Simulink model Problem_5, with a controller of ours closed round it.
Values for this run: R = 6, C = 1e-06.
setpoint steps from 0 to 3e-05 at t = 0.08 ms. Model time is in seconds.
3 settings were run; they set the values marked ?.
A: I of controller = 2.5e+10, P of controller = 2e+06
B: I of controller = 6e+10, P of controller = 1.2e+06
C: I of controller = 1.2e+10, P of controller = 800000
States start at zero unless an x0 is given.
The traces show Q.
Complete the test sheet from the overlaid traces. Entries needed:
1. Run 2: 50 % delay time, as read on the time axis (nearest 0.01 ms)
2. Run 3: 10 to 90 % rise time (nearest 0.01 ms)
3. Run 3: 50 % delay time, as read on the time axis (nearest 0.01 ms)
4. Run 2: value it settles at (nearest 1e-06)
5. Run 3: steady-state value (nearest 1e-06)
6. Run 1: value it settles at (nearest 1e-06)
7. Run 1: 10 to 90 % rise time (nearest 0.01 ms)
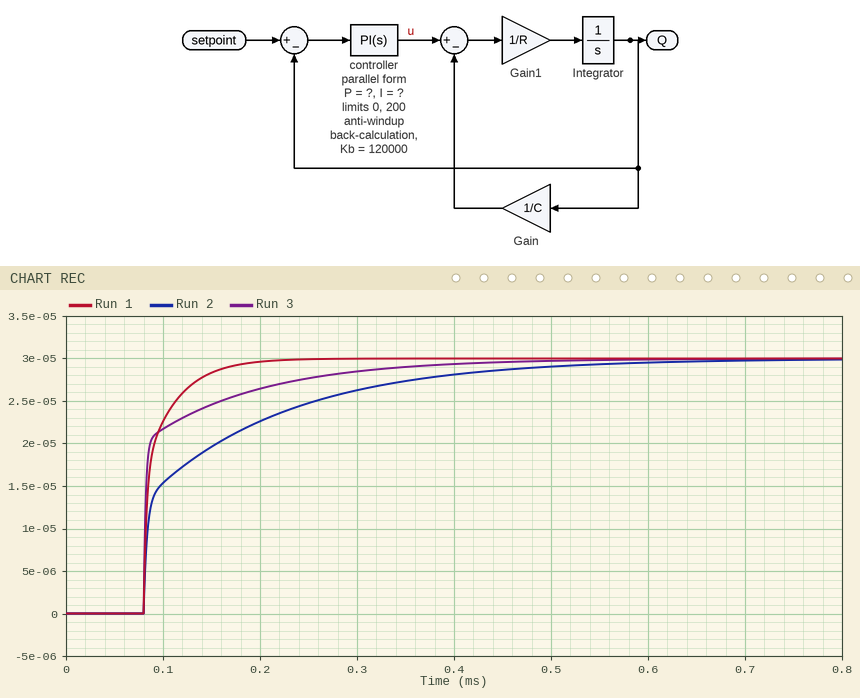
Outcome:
0.10 ms
0.14 ms
0.08 ms
0.000030
0.000030
0.000030
0.05 ms
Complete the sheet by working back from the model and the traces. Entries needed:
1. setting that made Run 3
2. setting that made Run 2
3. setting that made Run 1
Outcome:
A
C
B
